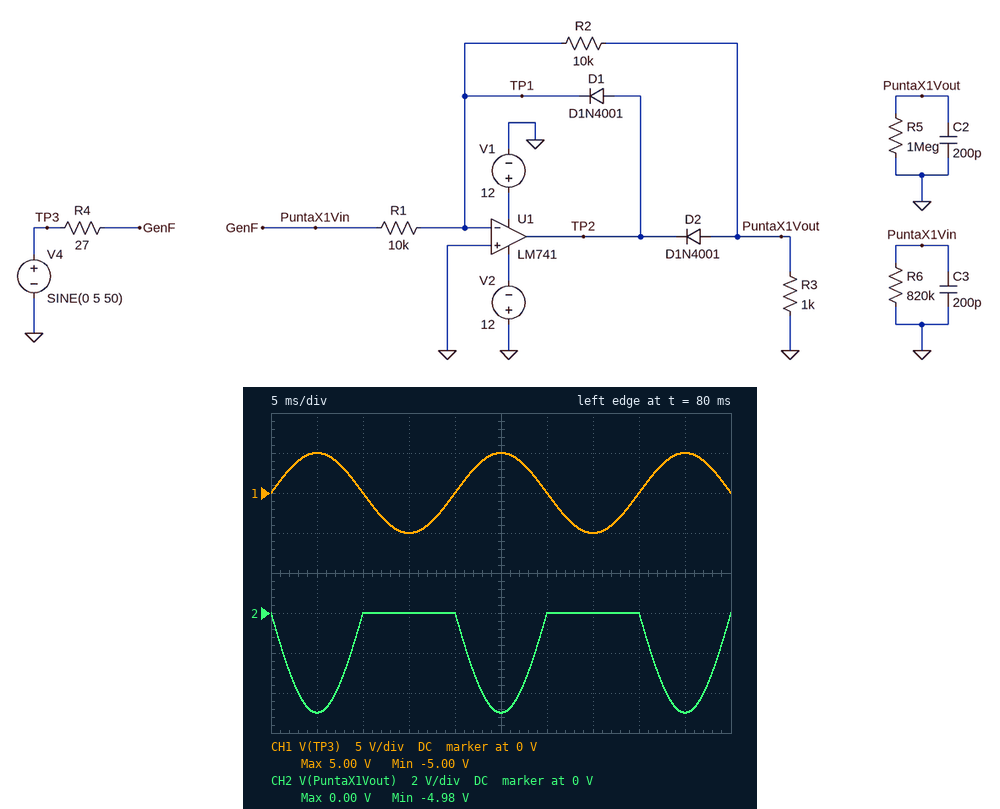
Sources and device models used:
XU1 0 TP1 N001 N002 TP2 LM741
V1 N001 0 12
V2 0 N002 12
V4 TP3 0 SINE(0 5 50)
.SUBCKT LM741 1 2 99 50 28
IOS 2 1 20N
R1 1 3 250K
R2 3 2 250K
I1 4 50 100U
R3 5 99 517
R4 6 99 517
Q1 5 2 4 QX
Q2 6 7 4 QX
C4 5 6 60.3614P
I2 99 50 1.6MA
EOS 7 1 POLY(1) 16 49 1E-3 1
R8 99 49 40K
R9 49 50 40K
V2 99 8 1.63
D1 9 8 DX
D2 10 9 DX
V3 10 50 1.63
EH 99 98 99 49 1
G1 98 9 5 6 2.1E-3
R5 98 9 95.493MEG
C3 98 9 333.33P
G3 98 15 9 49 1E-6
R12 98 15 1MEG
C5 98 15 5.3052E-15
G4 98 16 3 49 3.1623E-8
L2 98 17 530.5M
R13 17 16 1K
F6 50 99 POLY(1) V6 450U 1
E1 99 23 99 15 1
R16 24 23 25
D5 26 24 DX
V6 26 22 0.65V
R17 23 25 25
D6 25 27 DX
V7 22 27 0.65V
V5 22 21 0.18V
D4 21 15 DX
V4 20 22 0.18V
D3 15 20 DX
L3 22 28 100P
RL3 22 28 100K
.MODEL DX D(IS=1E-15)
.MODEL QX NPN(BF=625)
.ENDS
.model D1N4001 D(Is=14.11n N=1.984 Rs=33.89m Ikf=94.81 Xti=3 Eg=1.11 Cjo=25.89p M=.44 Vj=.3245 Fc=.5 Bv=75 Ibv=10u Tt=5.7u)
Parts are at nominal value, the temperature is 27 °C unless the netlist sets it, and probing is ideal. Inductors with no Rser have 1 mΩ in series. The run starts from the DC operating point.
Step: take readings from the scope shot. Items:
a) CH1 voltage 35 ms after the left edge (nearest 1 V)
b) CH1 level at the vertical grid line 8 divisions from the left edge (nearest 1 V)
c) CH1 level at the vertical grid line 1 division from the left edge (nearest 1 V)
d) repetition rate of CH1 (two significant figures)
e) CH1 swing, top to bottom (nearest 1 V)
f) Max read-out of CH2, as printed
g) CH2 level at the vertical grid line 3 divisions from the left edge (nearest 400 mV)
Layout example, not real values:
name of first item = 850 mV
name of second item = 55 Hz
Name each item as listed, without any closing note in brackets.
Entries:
CH1 voltage 35 ms after the left edge = -5 V
CH1 level at the vertical grid line 8 divisions from the left edge = 0 V
CH1 level at the vertical grid line 1 division from the left edge = 5 V
repetition rate of CH1 = 50 Hz
CH1 swing, top to bottom = 10 V
Max read-out of CH2, as printed = 0.00 V
CH2 level at the vertical grid line 3 divisions from the left edge = 0 V
